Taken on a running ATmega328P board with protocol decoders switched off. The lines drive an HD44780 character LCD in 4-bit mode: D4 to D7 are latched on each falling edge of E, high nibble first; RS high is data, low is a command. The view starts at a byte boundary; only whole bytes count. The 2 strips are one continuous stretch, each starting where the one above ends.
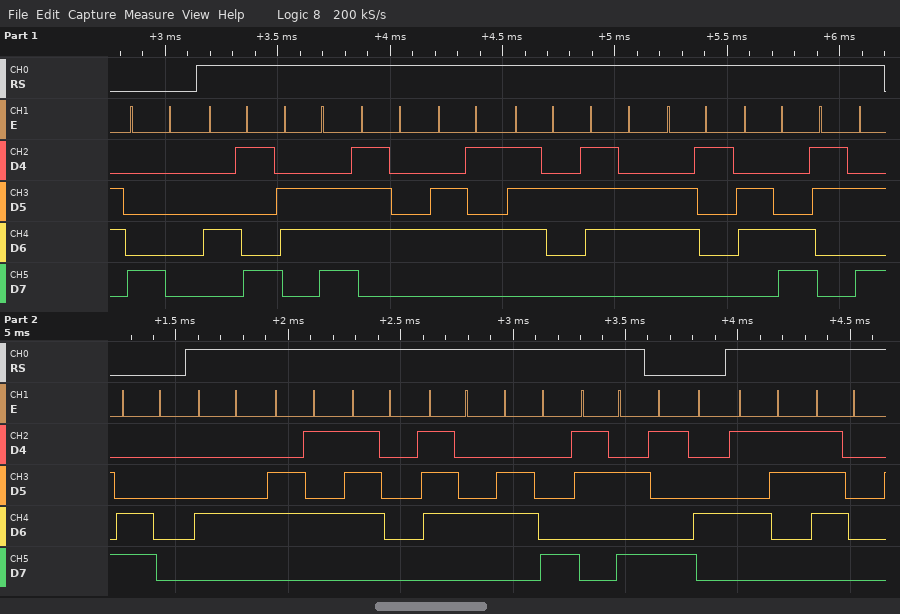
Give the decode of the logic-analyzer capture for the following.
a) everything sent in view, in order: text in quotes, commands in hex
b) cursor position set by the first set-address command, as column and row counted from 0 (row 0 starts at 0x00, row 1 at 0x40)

0x80 "Interval:" 0xC0 "Depth:" 0x94 "Sp"
column 0, row 0
